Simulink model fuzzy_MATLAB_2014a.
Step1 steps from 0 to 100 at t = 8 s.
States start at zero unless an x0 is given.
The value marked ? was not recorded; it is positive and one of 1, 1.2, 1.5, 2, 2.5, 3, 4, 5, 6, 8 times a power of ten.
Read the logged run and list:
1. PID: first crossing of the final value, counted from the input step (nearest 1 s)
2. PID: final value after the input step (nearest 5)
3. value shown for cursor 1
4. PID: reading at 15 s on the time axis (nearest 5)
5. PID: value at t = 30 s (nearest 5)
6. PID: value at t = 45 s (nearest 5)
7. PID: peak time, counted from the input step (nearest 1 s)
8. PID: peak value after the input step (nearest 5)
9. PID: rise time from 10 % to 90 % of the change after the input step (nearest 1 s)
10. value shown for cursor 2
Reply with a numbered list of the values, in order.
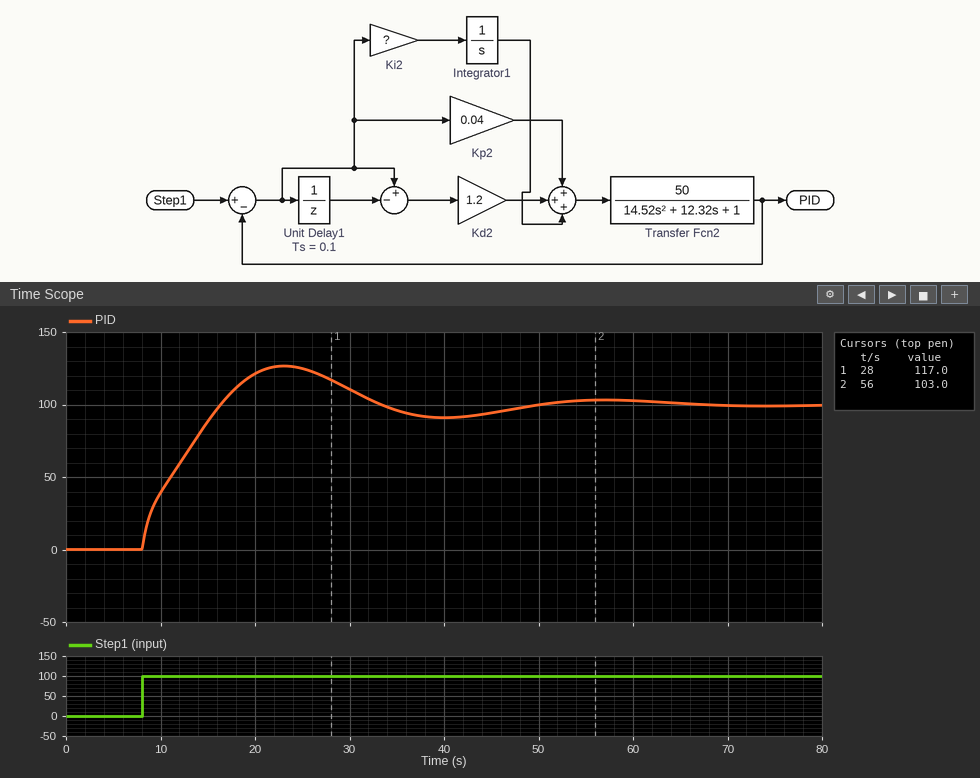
1. 8 s
2. 100
3. 117.0
4. 90
5. 110
6. 95
7. 15 s
8. 125
9. 7 s
10. 103.0
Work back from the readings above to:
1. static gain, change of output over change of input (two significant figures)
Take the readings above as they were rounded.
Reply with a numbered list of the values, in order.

1. 1.0
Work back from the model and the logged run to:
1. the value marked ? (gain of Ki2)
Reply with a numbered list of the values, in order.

1. 0.015
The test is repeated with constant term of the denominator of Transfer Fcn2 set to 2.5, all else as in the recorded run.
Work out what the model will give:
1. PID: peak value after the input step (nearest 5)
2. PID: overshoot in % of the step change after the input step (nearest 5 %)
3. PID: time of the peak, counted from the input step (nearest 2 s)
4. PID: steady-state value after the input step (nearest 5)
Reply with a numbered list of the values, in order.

1. 110
2. 10 %
3. 18 s
4. 100
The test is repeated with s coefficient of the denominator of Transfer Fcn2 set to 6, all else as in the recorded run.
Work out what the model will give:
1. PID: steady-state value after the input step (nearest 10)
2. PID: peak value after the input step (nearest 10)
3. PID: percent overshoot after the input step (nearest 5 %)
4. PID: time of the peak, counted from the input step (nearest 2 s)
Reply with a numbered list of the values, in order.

1. 100
2. 120
3. 20 %
4. 12 s
